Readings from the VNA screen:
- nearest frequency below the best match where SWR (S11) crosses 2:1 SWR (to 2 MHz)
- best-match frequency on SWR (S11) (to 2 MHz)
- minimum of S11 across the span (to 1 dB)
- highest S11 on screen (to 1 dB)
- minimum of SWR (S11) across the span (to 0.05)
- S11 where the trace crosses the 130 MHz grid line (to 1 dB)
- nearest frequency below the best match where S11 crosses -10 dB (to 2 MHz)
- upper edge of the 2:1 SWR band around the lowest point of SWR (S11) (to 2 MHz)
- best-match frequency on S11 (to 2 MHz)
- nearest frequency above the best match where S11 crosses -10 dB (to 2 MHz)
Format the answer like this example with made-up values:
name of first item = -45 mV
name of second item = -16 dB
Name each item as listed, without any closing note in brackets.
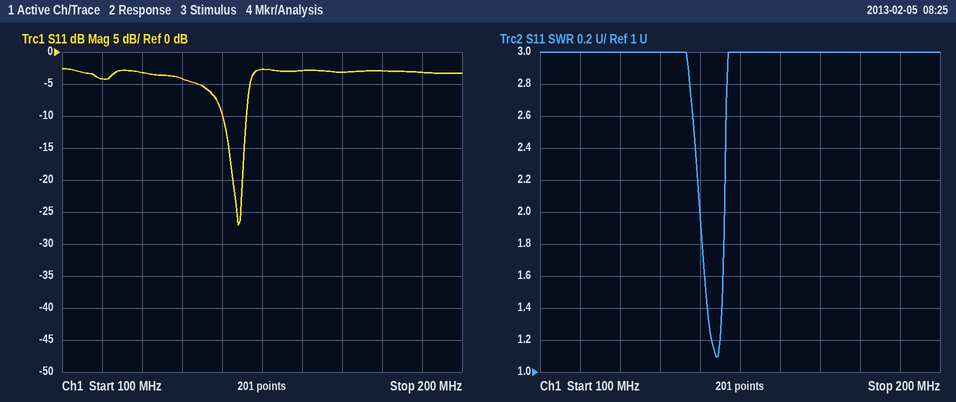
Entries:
nearest frequency below the best match where SWR (S11) crosses 2:1 SWR = 140 MHz
best-match frequency on SWR (S11) = 144 MHz
minimum of S11 across the span = -27 dB
highest S11 on screen = -3 dB
minimum of SWR (S11) across the span = 1.10
S11 where the trace crosses the 130 MHz grid line = -4 dB
nearest frequency below the best match where S11 crosses -10 dB = 140 MHz
upper edge of the 2:1 SWR band around the lowest point of SWR (S11) = 146 MHz
best-match frequency on S11 = 144 MHz
nearest frequency above the best match where S11 crosses -10 dB = 146 MHz
